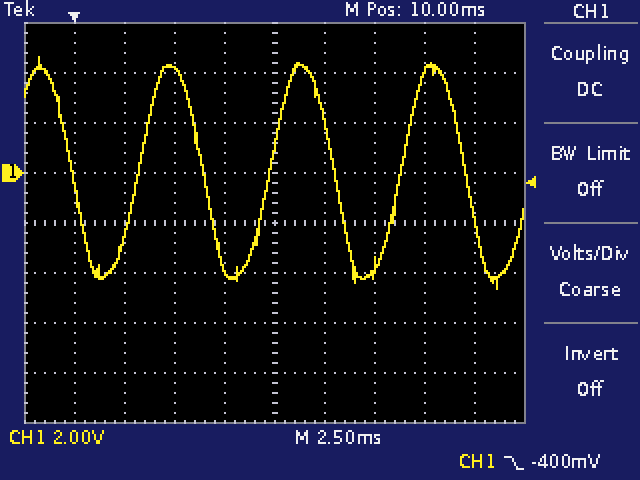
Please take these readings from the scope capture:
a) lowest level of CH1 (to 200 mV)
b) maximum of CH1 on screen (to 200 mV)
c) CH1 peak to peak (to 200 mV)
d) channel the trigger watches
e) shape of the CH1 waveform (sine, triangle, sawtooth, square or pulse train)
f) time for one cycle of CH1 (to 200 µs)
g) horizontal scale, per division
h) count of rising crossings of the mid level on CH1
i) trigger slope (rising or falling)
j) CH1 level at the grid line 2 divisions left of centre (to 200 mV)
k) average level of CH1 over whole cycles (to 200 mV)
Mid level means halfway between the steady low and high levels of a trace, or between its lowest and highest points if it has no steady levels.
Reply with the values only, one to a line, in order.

-4.6 V
4.6 V
9.2 V
CH1
sine
6.6 ms
2.5 ms
3
falling
4.2 V
0.0 V
